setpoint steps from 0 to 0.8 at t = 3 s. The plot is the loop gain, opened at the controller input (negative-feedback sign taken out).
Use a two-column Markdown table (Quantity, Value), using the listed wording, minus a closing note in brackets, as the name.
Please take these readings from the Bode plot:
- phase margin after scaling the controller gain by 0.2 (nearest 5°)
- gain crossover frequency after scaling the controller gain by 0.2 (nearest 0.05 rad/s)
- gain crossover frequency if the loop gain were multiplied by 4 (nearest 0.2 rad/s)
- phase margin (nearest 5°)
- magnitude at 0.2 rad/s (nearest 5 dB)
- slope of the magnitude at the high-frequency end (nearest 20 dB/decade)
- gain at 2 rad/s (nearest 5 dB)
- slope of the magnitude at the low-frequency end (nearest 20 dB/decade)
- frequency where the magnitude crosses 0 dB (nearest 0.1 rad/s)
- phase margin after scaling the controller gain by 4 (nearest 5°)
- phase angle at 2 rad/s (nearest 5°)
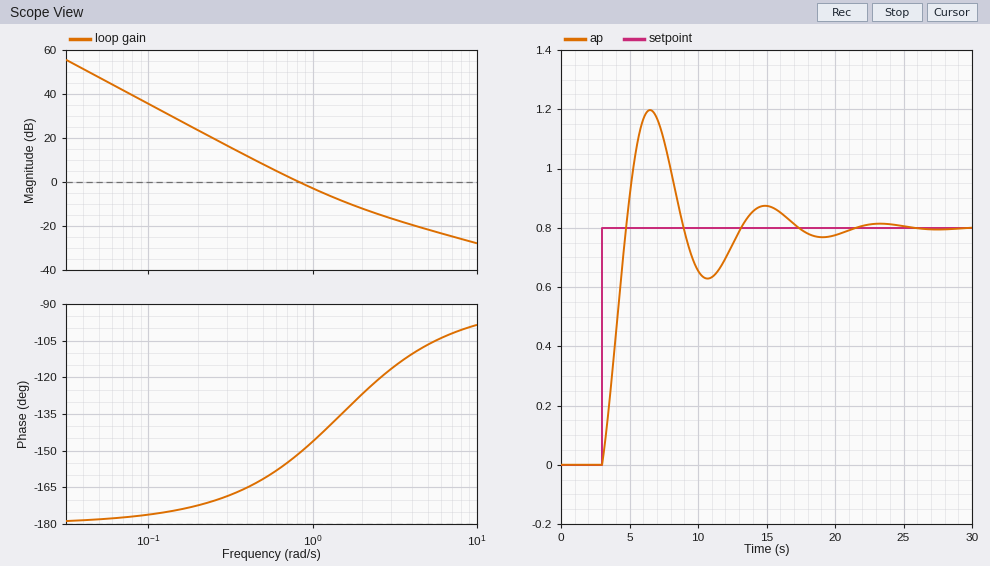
| Quantity | Value |
|---|---|
| phase margin after scaling the controller gain by 0.2 | 15° |
| gain crossover frequency after scaling the controller gain by 0.2 | 0.35 rad/s |
| gain crossover frequency if the loop gain were multiplied by 4 | 2.0 rad/s |
| phase margin | 30° |
| magnitude at 0.2 rad/s | 25 dB |
| slope of the magnitude at the high-frequency end | -20 dB/decade |
| gain at 2 rad/s | -10 dB |
| slope of the magnitude at the low-frequency end | -40 dB/decade |
| frequency where the magnitude crosses 0 dB | 0.8 rad/s |
| phase margin after scaling the controller gain by 4 | 55° |
| phase angle at 2 rad/s | -125° |
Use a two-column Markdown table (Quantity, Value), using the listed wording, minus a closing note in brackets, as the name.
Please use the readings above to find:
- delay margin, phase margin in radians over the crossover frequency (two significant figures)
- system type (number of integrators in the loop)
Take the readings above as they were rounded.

| Quantity | Value |
|---|---|
| delay margin, phase margin in radians over the crossover frequency | 0.65 s |
| system type | 2 |
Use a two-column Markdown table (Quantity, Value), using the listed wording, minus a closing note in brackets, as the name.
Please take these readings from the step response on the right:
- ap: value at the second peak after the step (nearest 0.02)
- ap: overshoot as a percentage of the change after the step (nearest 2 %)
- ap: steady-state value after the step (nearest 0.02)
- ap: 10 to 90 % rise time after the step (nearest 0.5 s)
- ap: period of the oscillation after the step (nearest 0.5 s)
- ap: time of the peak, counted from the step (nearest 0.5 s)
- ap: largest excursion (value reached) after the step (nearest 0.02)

| Quantity | Value |
|---|---|
| ap: value at the second peak after the step | 0.88 |
| ap: overshoot as a percentage of the change after the step | 50 % |
| ap: steady-state value after the step | 0.80 |
| ap: 10 to 90 % rise time after the step | 1.5 s |
| ap: period of the oscillation after the step | 8.5 s |
| ap: time of the peak, counted from the step | 3.5 s |
| ap: largest excursion (value reached) after the step | 1.20 |
